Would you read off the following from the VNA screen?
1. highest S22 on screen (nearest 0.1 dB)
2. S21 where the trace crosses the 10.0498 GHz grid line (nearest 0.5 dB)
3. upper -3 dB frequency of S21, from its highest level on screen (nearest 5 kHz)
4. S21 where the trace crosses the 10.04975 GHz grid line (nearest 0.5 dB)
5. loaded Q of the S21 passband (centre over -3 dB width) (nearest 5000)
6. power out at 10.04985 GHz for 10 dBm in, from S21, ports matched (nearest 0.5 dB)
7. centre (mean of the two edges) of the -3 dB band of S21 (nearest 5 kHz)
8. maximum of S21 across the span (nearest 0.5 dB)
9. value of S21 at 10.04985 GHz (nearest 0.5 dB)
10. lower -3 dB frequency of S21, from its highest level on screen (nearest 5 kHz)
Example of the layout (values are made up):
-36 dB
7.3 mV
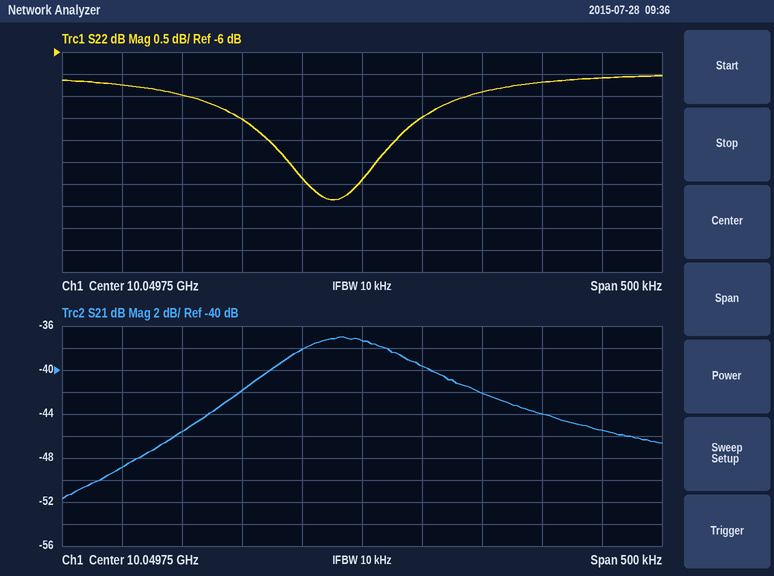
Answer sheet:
-6.5 dB
-39.5 dB
10.049805 GHz
-37.5 dB
75000
-32.0 dBm
10.049740 GHz
-37.0 dB
-42.0 dB
10.049675 GHz
